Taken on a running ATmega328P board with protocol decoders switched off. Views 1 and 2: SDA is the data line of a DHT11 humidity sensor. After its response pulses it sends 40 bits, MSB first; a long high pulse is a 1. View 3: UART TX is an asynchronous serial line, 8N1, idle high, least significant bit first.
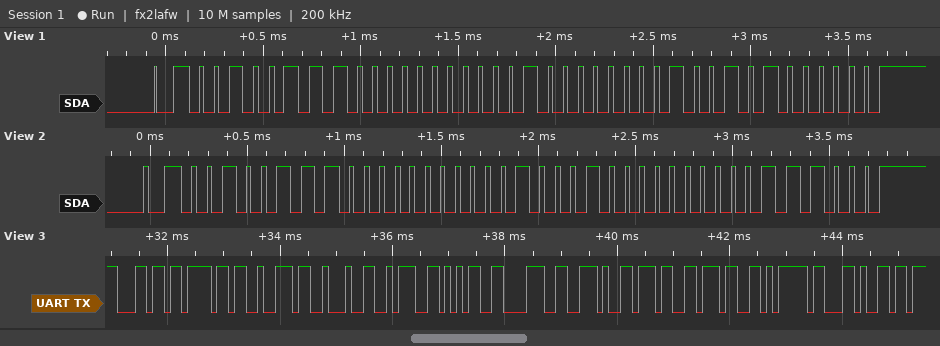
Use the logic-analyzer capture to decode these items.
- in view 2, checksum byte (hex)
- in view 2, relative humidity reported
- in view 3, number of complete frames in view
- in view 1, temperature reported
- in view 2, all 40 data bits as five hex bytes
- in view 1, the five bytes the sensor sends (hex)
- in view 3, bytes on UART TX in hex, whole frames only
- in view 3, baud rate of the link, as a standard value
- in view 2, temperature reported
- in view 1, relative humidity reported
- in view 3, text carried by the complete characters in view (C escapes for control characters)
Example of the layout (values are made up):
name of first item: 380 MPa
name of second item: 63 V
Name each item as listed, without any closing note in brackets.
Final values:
in view 2, checksum byte: 0x38
in view 2, relative humidity reported: 39 %
in view 3, number of complete frames in view: 12
in view 1, temperature reported: 16.9 °C
in view 2, all 40 data bits as five hex bytes: 27 00 11 00 38
in view 1, the five bytes the sensor sends: 27 00 10 09 40
in view 3, bytes on UART TX in hex, whole frames only: 6C 6F 72 22 3A 35 38 2E 37 37 7D 2C
in view 3, baud rate of the link, as a standard value: 9600 baud
in view 2, temperature reported: 17.0 °C
in view 1, relative humidity reported: 39 %
in view 3, text carried by the complete characters in view: "lor\":58.77},"
